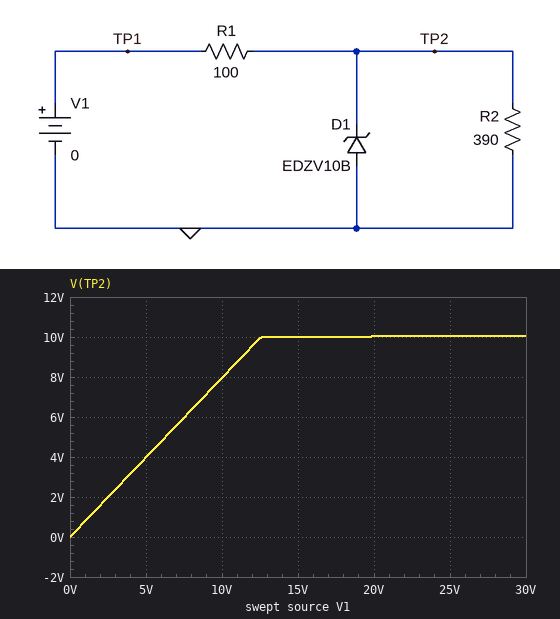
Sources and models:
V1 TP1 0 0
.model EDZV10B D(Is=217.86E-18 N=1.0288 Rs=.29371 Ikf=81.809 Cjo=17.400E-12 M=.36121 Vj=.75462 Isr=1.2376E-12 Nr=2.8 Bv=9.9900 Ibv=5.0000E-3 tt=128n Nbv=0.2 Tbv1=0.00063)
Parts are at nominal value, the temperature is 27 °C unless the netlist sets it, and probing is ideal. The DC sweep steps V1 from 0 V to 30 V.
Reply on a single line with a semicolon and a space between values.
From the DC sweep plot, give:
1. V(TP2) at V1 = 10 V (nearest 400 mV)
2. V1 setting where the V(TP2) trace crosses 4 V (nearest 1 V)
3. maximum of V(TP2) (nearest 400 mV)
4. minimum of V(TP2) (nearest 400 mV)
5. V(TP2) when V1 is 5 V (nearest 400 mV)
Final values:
8.0 V; 5 V; 10.0 V; 0 V; 4.0 V
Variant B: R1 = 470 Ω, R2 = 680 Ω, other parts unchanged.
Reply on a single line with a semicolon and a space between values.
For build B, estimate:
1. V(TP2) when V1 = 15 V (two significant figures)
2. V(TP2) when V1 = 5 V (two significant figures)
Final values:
8.9 V; 3.0 V
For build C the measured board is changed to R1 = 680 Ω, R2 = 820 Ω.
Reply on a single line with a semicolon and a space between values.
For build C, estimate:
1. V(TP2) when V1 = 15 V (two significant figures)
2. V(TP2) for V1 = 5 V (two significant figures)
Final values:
8.2 V; 2.7 V
